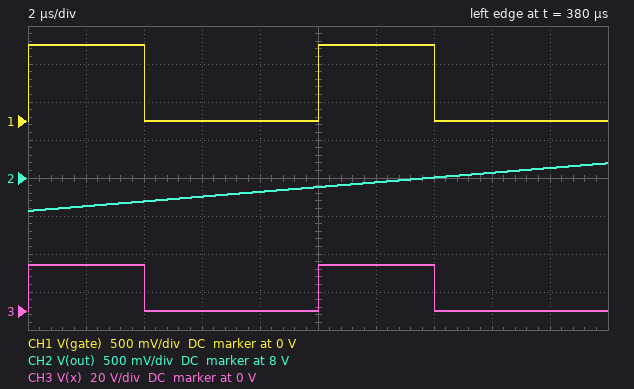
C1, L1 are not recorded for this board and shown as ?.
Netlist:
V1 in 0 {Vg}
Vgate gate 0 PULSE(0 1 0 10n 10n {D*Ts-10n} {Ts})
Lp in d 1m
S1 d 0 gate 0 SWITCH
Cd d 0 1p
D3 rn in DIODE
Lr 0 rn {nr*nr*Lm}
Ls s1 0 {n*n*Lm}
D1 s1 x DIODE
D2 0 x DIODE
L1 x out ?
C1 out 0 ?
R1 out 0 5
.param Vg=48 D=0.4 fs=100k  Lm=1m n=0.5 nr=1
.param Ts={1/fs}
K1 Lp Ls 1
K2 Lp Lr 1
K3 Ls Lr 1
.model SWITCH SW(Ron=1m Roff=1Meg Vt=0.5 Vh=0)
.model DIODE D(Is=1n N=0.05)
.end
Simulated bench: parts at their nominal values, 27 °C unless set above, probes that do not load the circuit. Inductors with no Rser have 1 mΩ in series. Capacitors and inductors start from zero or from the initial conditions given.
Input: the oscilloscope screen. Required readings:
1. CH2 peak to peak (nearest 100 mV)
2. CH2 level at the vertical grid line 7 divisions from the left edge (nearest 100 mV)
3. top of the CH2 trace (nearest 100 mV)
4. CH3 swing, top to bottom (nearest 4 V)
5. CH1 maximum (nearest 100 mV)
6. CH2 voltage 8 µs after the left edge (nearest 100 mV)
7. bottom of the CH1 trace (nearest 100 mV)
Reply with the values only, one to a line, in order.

600 mV
8.0 V
8.2 V
24 V
1.0 V
7.8 V
0 V
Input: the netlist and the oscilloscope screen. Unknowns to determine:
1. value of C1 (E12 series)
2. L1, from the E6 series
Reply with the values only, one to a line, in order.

330 µF
220 µH
